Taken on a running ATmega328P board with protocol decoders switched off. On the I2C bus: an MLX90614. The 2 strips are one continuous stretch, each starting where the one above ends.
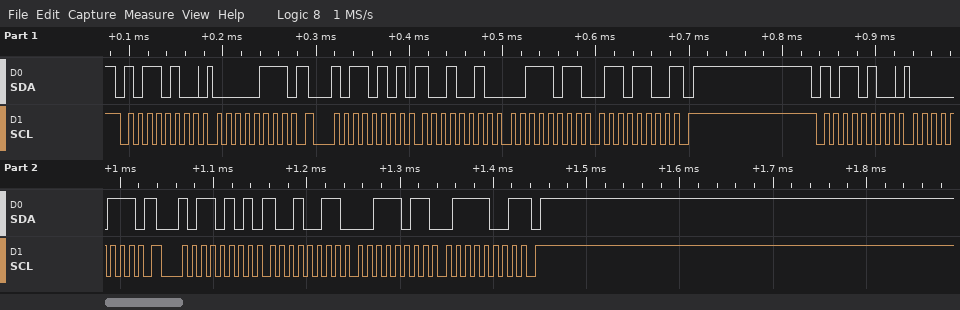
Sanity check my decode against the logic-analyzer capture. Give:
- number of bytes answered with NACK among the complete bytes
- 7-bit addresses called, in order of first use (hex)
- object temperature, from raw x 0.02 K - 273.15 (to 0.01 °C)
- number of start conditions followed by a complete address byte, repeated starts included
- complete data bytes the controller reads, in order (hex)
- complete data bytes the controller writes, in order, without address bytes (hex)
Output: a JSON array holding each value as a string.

["2", "0x5A", "31.85 °C", "4", "92 3B 6C 93 3B 79", "07 07"]
